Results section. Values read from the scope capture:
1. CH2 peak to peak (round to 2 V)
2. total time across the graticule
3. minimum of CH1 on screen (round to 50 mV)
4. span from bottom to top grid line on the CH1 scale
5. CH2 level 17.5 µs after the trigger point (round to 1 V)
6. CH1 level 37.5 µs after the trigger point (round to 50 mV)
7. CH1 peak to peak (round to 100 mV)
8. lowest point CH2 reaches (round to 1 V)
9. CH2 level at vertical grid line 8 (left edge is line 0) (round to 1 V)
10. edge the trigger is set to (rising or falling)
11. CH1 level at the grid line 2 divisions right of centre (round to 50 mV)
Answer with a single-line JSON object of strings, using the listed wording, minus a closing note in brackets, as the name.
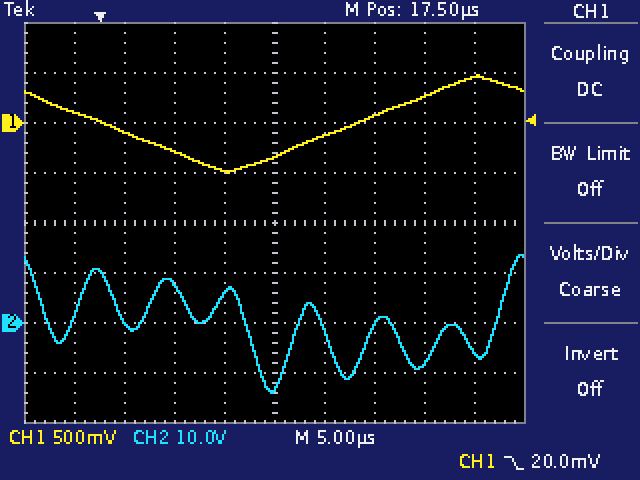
{"CH2 peak to peak": "28 V", "total time across the graticule": "50 µs", "minimum of CH1 on screen": "-500 mV", "span from bottom to top grid line on the CH1 scale": "4 V", "CH2 level 17.5 µs after the trigger point": "-13 V", "CH1 level 37.5 µs after the trigger point": "450 mV", "CH1 peak to peak": "1.00 V", "lowest point CH2 reaches": "-14 V", "CH2 level at vertical grid line 8 (left edge is line 0)": "-8 V", "edge the trigger is set to": "falling", "CH1 level at the grid line 2 divisions right of centre": "50 mV"}
